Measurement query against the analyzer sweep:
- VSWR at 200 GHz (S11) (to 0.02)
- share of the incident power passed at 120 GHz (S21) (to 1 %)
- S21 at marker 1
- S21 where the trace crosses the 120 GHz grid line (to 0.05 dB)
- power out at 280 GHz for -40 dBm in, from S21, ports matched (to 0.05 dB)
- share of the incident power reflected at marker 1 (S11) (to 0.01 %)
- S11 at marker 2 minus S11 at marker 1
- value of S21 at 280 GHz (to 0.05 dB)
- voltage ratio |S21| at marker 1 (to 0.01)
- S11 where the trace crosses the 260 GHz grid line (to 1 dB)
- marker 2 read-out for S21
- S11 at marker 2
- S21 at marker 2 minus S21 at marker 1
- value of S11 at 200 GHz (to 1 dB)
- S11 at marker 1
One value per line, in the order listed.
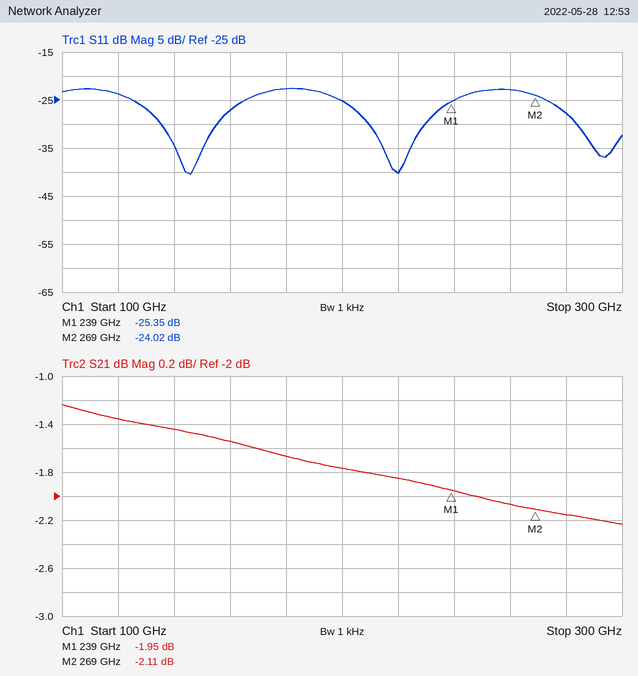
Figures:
1.12
73 %
-1.95 dB
-1.35 dB
-42.15 dBm
0.29 %
1.33 dB
-2.15 dB
0.80
-23 dB
-2.11 dB
-24.02 dB
-0.16 dB
-25 dB
-25.35 dB
